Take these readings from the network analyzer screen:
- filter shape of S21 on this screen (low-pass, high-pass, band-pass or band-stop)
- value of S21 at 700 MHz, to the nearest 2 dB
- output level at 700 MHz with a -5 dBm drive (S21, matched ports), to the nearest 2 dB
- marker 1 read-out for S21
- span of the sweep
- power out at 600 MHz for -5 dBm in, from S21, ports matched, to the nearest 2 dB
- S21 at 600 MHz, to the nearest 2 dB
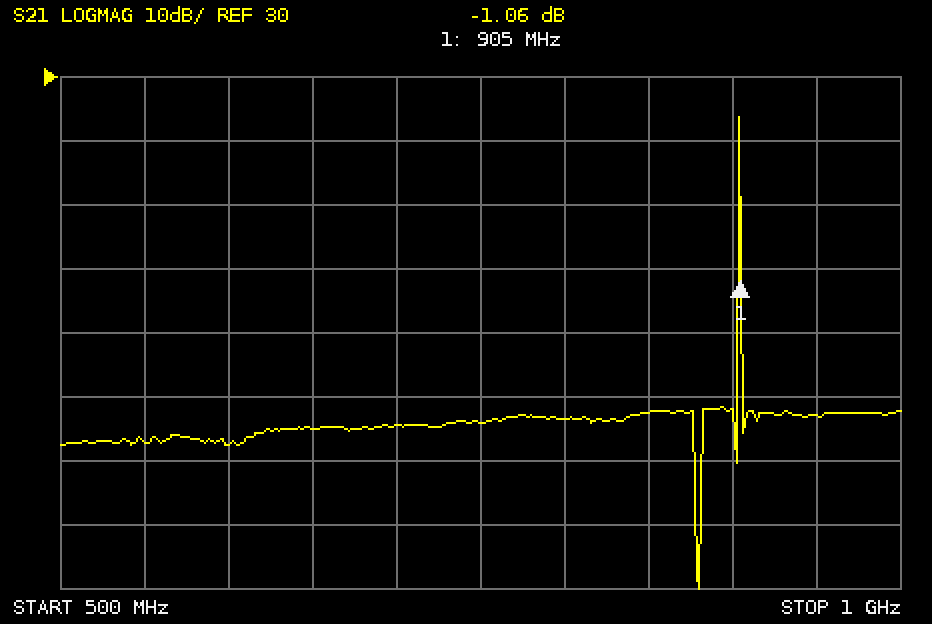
band-pass
-24 dB
-30 dBm
-1.06 dB
500 MHz
-32 dBm
-28 dB
